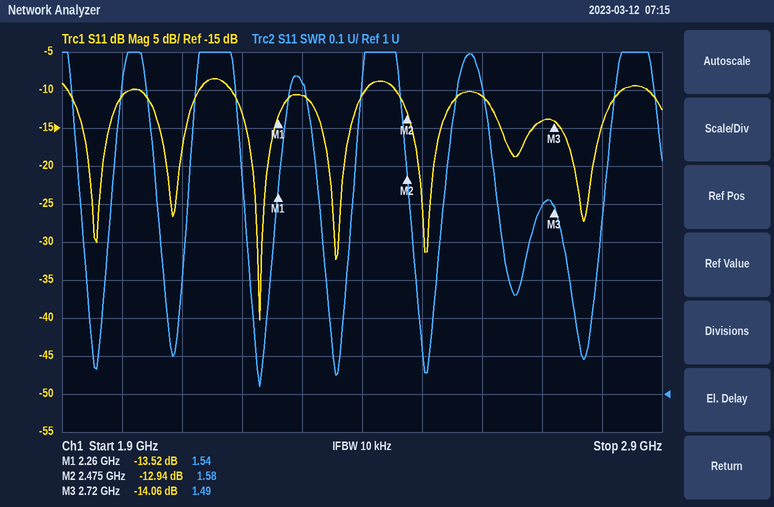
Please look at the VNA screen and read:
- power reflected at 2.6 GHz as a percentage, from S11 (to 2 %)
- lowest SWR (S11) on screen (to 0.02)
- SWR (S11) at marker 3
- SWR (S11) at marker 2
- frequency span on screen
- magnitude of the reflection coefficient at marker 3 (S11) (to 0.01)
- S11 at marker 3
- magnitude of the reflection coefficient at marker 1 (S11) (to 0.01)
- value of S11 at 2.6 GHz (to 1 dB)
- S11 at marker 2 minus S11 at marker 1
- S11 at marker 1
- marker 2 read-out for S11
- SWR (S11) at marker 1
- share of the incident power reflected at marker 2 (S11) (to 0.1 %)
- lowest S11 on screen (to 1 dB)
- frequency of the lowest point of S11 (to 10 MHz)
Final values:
8 %
1.02
1.49
1.58
1 GHz
0.20
-14.06 dB
0.21
-11 dB
0.58 dB
-13.52 dB
-12.94 dB
1.54
5.1 %
-40 dB
2.23 GHz
